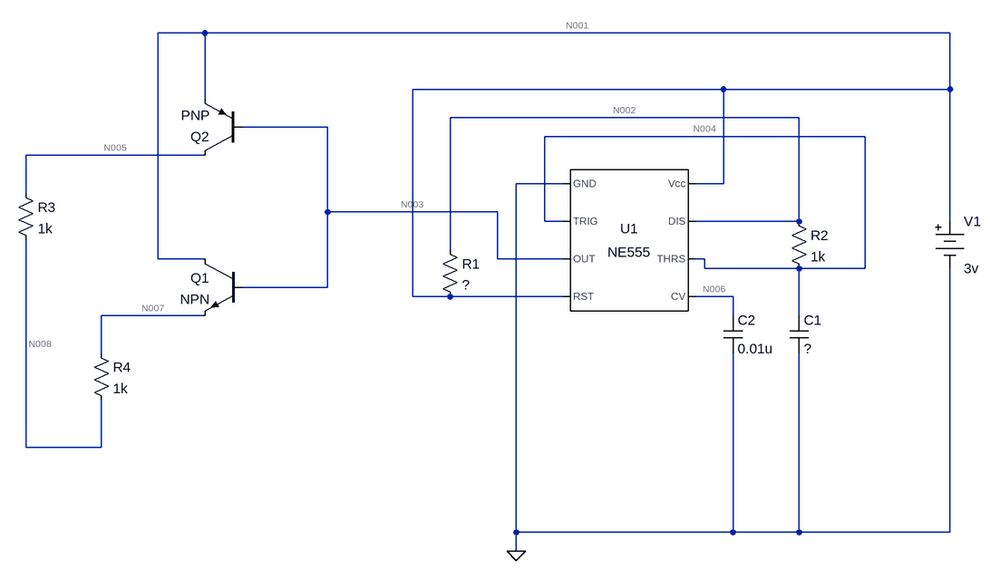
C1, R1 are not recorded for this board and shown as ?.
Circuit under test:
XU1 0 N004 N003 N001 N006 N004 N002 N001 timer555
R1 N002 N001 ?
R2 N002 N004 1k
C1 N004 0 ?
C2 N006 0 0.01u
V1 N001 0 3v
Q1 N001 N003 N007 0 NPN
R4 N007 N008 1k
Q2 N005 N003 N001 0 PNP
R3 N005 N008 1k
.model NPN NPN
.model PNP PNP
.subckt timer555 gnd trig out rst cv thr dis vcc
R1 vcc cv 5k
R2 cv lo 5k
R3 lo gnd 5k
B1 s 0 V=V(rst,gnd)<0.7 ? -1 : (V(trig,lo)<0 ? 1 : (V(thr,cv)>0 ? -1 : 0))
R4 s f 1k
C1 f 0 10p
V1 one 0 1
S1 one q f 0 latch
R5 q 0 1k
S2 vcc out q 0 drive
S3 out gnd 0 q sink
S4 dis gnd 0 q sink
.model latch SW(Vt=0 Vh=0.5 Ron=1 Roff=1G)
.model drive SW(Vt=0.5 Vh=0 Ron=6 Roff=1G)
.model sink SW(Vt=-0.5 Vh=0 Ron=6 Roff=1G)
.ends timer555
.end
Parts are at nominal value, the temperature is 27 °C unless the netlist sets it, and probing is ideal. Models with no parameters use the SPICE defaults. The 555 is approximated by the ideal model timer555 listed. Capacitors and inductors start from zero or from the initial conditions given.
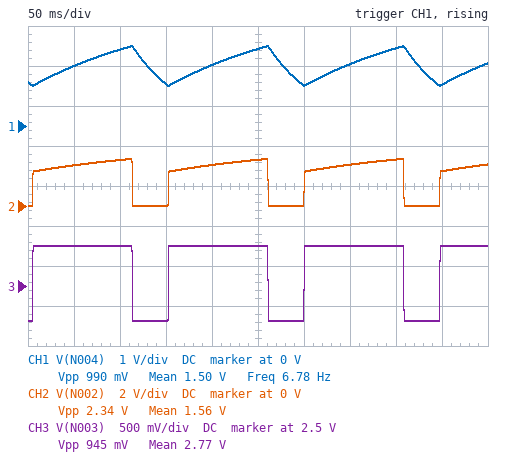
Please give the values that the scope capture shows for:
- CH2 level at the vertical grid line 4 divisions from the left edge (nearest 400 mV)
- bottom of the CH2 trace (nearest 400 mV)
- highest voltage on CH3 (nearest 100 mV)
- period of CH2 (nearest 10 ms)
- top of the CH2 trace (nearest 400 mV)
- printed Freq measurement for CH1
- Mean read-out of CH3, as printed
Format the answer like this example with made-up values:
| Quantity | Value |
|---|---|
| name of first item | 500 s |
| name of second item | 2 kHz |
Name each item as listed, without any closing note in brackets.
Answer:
| Quantity | Value |
|---|---|
| CH2 level at the vertical grid line 4 divisions from the left edge | 2.0 V |
| bottom of the CH2 trace | 0 V |
| highest voltage on CH3 | 3.0 V |
| period of CH2 | 150 ms |
| top of the CH2 trace | 2.4 V |
| printed Freq measurement for CH1 | 6.78 Hz |
| Mean read-out of CH3, as printed | 2.77 V |
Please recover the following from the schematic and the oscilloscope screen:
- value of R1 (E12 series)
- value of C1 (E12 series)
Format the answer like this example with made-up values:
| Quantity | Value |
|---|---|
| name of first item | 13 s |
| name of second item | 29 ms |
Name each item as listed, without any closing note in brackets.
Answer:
| Quantity | Value |
|---|---|
| value of R1 | 1.8 kΩ |
| value of C1 | 56 µF |
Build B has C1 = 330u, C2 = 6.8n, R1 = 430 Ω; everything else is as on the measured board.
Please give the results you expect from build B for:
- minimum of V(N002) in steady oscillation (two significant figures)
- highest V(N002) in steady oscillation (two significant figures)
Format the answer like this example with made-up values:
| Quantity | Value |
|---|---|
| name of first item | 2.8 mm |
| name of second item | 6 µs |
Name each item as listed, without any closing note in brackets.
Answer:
| Quantity | Value |
|---|---|
| minimum of V(N002) in steady oscillation | 47 mV |
| highest V(N002) in steady oscillation | 2.7 V |
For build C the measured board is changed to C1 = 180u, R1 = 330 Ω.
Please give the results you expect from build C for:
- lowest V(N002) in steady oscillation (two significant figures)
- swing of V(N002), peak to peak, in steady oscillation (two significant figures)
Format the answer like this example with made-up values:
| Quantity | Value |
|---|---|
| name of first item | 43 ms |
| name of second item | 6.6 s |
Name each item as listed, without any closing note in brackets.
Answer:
| Quantity | Value |
|---|---|
| lowest V(N002) in steady oscillation | 59 mV |
| swing of V(N002), peak to peak, in steady oscillation | 2.7 V |
